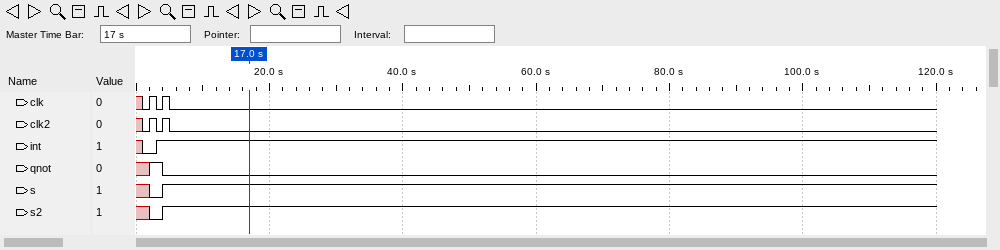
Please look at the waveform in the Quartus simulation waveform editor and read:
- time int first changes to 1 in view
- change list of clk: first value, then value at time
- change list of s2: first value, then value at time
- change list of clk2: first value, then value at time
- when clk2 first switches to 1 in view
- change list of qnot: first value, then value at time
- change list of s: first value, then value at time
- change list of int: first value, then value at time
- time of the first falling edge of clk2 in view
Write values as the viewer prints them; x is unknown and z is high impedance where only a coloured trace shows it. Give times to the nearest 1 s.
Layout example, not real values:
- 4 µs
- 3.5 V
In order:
- 3 s
- x, 0 at 1 s, 1 at 2 s, 0 at 3 s, 1 at 4 s, 0 at 5 s
- x, 0 at 2 s, 1 at 4 s
- x, 0 at 1 s, 1 at 2 s, 0 at 3 s, 1 at 4 s, 0 at 5 s
- 2 s
- x, 1 at 2 s, 0 at 4 s
- x, 0 at 2 s, 1 at 4 s
- x, 0 at 1 s, 1 at 3 s
- 3 s
